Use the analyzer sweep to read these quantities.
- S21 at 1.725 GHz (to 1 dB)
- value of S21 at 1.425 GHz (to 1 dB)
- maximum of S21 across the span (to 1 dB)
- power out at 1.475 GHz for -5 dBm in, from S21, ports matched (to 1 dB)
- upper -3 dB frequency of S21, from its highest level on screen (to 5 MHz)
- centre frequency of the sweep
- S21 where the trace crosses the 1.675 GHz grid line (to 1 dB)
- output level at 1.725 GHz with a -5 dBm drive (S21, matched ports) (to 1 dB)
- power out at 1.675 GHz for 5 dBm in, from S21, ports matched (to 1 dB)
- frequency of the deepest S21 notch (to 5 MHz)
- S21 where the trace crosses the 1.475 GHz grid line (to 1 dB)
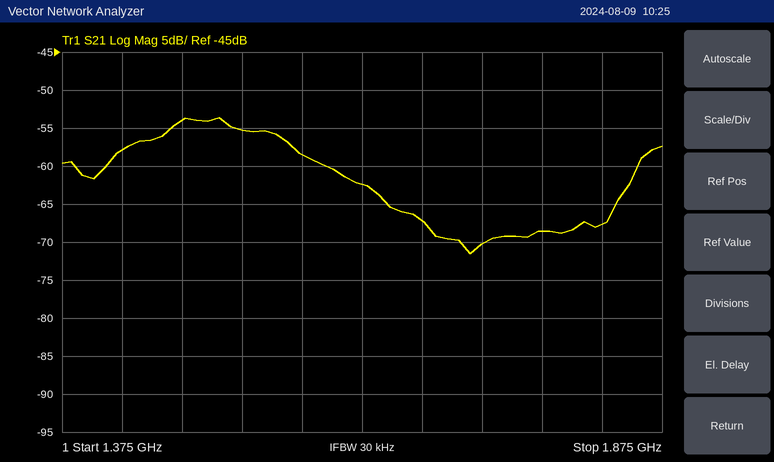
-70 dB
-58 dB
-54 dB
-59 dBm
1.560 GHz
1.625 GHz
-67 dB
-75 dBm
-62 dBm
1.715 GHz
-54 dB
